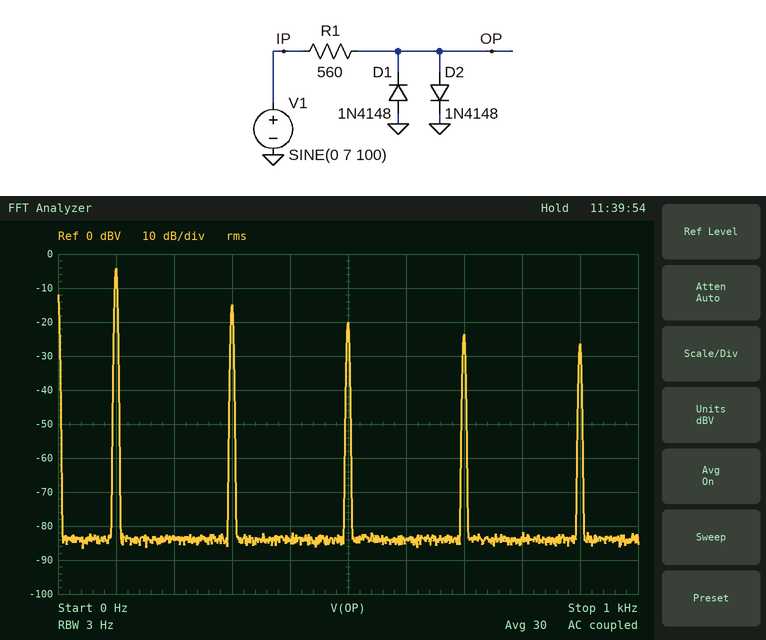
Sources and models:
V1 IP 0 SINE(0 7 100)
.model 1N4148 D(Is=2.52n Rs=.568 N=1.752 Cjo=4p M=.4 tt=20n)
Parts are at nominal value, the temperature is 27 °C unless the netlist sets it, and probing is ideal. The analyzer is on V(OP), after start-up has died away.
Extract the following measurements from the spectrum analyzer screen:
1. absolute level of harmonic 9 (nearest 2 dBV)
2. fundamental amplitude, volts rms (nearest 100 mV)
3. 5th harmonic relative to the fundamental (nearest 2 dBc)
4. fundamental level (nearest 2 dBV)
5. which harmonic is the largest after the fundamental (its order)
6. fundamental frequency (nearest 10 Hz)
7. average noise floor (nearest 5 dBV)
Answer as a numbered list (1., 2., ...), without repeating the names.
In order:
1. -26 dBV
2. 600 mV
3. -16 dBc
4. -4 dBV
5. 3
6. 100 Hz
7. -85 dBV
